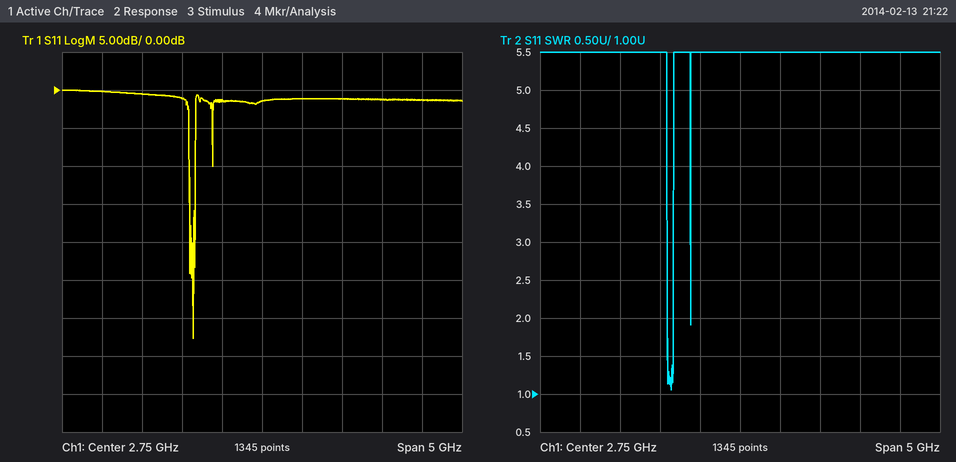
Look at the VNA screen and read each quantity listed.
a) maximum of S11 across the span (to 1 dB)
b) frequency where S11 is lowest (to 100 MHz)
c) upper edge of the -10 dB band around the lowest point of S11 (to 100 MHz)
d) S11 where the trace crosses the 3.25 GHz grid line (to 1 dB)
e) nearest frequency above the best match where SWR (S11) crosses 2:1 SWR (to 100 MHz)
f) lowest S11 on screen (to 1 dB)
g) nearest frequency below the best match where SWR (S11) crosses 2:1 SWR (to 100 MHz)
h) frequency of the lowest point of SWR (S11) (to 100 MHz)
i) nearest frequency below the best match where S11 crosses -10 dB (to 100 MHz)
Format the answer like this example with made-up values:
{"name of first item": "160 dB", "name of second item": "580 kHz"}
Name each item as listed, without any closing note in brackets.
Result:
{"maximum of S11 across the span": "0 dB", "frequency where S11 is lowest": "1.9 GHz", "upper edge of the -10 dB band around the lowest point of S11": "1.9 GHz", "S11 where the trace crosses the 3.25 GHz grid line": "-1 dB", "nearest frequency above the best match where SWR (S11) crosses 2:1 SWR": "1.9 GHz", "lowest S11 on screen": "-33 dB", "nearest frequency below the best match where SWR (S11) crosses 2:1 SWR": "1.8 GHz", "frequency of the lowest point of SWR (S11)": "1.9 GHz", "nearest frequency below the best match where S11 crosses -10 dB": "1.8 GHz"}
